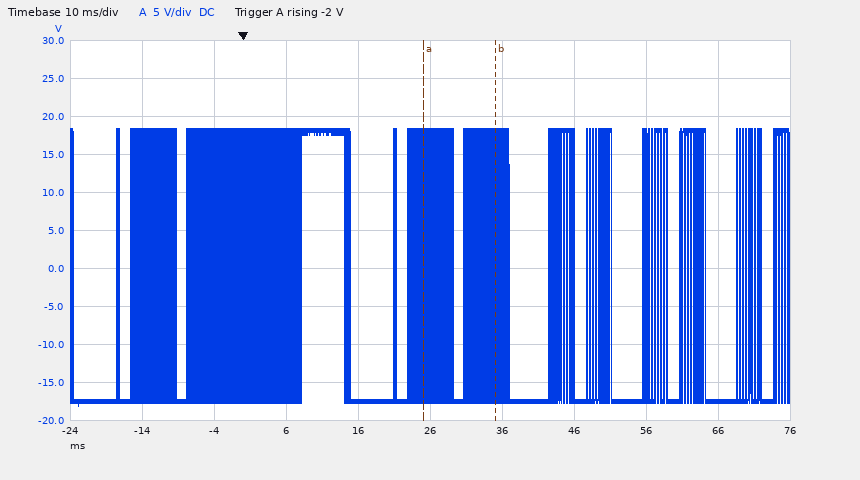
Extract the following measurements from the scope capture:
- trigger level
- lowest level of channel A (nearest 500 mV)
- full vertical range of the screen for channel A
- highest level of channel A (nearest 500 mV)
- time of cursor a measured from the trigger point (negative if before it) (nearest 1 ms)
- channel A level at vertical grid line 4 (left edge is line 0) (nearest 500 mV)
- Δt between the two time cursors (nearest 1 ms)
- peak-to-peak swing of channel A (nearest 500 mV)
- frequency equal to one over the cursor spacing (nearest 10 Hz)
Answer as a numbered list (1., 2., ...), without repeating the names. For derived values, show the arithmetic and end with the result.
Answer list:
1. -2 V
2. -18.0 V
3. 50 V
4. 18.5 V
5. +25 ms
6. -17.5 V
7. 10 ms
8. 18.5 V − (-18.0 V) = 36.5 V
9. 1 / 10 ms ≈ 100 Hz
